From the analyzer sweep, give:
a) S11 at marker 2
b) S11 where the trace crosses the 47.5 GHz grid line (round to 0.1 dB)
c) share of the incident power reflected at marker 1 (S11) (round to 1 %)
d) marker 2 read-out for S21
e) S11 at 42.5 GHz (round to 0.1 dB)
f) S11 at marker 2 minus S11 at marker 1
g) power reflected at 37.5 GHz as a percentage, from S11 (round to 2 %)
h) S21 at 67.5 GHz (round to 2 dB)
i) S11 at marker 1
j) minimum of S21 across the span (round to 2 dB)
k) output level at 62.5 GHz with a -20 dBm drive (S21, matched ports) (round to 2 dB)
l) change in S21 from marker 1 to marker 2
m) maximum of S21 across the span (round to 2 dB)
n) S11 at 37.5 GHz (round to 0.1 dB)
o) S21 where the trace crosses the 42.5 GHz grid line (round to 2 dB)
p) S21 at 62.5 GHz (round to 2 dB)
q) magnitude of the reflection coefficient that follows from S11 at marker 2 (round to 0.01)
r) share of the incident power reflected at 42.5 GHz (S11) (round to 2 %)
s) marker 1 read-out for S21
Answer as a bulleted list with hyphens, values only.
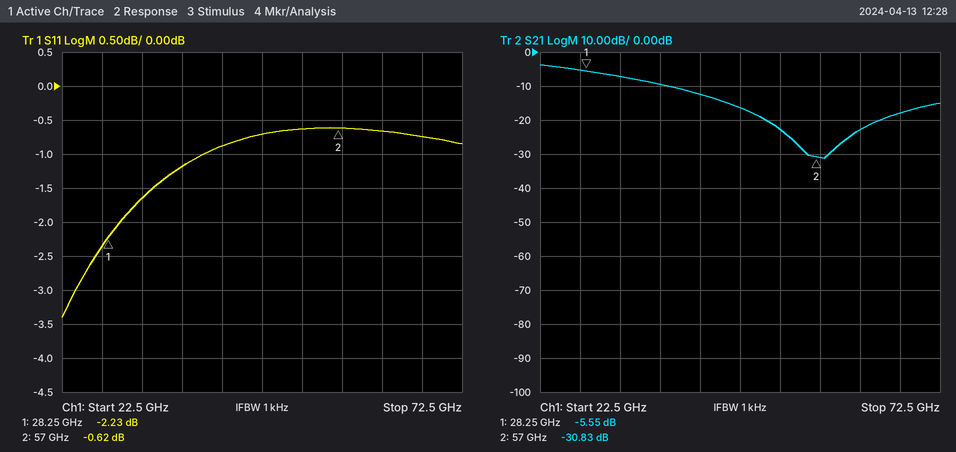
- -0.62 dB
- -0.7 dB
- 60 %
- -30.83 dB
- -0.9 dB
- 1.61 dB
- 76 %
- -18 dB
- -2.23 dB
- -32 dB
- -42 dBm
- -25.28 dB
- -4 dB
- -1.2 dB
- -12 dB
- -22 dB
- 0.93
- 82 %
- -5.55 dB
